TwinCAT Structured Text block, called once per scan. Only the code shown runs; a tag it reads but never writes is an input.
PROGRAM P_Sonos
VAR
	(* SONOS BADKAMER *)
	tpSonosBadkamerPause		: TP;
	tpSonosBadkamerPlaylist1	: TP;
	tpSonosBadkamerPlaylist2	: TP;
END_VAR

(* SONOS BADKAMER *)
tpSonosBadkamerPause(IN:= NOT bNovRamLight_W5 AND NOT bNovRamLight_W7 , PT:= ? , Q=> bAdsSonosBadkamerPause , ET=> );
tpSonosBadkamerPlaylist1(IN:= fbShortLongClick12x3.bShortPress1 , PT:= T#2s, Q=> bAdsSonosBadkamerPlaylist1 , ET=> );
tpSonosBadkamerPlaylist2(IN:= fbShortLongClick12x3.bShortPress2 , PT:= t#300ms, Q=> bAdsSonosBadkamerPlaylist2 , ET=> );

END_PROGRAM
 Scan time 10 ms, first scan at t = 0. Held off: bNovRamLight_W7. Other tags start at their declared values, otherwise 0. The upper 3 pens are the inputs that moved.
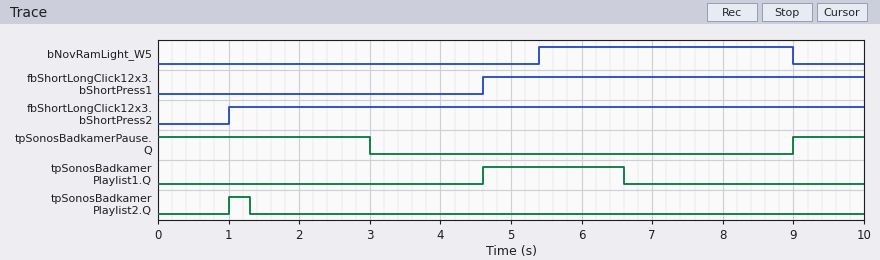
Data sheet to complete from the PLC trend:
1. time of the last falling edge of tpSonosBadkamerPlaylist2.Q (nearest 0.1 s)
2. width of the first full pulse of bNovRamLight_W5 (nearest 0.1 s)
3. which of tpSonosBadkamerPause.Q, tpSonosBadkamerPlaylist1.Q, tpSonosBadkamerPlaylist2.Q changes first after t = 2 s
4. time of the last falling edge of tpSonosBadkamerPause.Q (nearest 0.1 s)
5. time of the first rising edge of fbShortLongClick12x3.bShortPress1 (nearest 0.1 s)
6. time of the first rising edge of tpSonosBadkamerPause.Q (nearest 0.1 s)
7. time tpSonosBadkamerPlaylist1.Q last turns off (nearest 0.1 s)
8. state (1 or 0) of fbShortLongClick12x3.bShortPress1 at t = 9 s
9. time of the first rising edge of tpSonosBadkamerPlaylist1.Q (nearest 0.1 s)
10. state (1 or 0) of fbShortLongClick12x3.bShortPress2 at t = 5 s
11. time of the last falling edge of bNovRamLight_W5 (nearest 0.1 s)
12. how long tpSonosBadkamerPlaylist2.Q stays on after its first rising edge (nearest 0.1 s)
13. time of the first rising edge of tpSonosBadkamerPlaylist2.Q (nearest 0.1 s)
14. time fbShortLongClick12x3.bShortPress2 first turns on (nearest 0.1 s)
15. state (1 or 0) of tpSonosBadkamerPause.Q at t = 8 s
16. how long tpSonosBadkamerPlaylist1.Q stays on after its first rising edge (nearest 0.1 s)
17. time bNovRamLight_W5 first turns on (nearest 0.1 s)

1.3 s
3.6 s
tpSonosBadkamerPause.Q
3.0 s
4.6 s
9.0 s
6.6 s
1
4.6 s
1
9.0 s
0.3 s
1.0 s
1.0 s
0
2.0 s
5.4 s
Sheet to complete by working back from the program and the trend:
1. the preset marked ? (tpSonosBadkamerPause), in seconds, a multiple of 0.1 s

3.0 s
